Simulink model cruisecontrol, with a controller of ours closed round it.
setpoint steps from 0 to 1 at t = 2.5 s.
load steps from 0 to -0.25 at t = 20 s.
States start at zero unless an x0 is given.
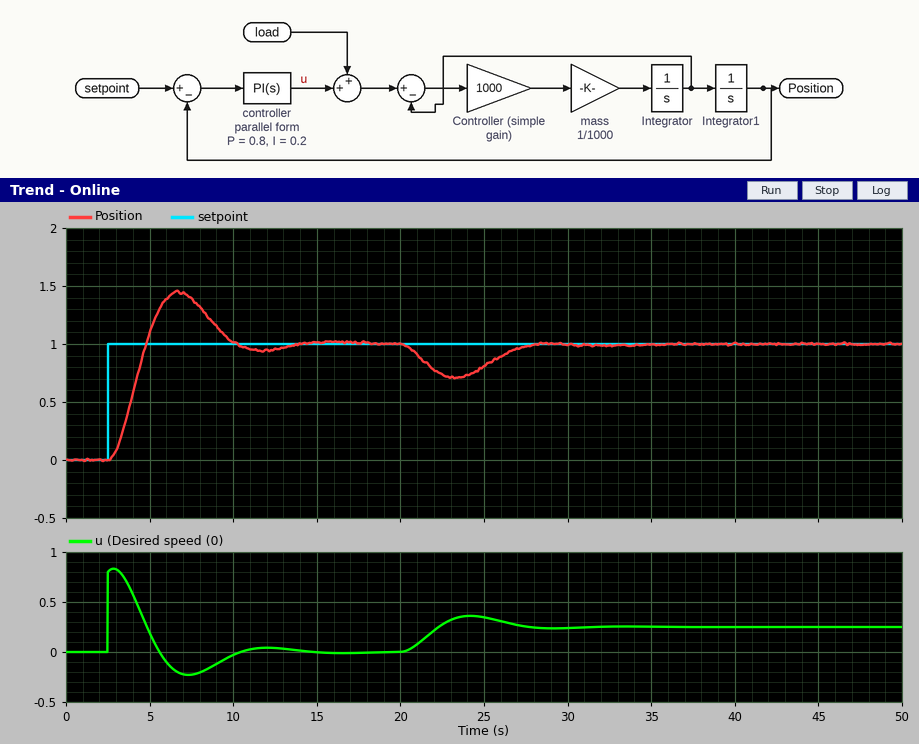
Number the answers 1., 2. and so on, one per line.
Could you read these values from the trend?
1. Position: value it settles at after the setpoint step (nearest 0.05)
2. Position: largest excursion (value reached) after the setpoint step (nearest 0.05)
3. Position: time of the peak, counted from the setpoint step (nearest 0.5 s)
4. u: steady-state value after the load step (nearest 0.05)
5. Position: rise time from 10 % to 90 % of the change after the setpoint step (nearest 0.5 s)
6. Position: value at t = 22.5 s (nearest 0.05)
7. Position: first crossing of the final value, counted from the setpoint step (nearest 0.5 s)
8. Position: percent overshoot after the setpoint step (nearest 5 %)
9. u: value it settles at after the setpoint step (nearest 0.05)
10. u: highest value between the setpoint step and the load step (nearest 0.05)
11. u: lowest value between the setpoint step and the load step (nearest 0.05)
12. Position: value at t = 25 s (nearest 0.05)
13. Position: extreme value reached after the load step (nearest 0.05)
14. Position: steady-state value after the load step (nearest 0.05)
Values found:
1. 1.00
2. 1.45
3. 4.0 s
4. 0.25
5. 1.5 s
6. 0.75
7. 2.5 s
8. 45 %
9. 0.00
10. 0.85
11. -0.25
12. 0.80
13. 0.70
14. 1.00
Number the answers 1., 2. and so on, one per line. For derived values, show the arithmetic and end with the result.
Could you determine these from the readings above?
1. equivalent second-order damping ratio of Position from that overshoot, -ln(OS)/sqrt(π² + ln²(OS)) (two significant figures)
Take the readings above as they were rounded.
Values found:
1. ln(0.45) = -0.799; 0.799 / sqrt(9.870 + 0.638) = 0.25
